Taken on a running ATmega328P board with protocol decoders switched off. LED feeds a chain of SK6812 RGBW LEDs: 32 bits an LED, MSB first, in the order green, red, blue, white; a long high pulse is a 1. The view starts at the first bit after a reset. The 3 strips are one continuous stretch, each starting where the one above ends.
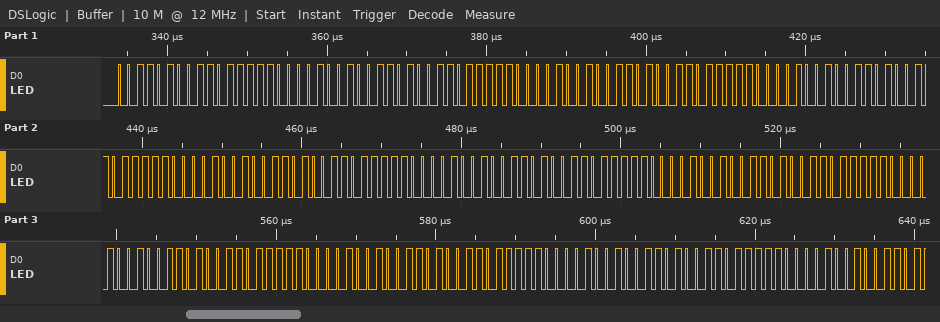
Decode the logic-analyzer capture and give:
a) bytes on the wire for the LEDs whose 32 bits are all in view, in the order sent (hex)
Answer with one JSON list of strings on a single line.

["34 DF 09 34 DF 09 34 DF 09 34 DF 09 34 DF 09 34 DF 09 34 DF 09 34 DF 09 34 DF 09 34"]
